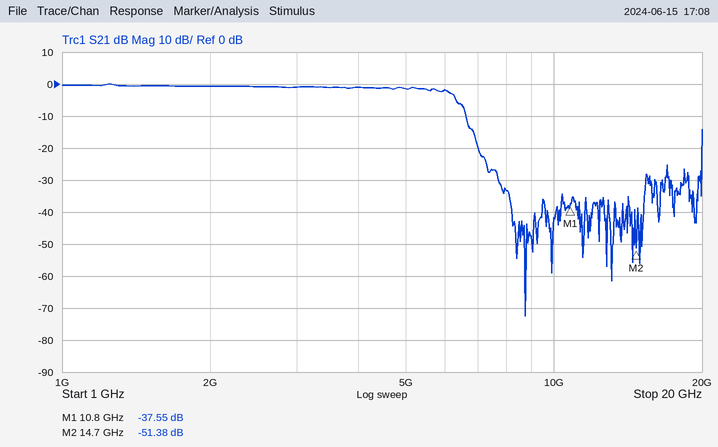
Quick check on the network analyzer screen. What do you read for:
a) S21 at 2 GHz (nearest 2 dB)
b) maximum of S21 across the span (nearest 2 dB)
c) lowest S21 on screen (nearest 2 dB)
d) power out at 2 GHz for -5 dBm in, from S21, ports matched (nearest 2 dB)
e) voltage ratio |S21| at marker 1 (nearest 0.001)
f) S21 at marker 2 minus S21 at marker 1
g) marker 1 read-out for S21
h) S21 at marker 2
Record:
0 dB
0 dB
-72 dB
-6 dBm
0.013
-13.83 dB
-37.55 dB
-51.38 dB
